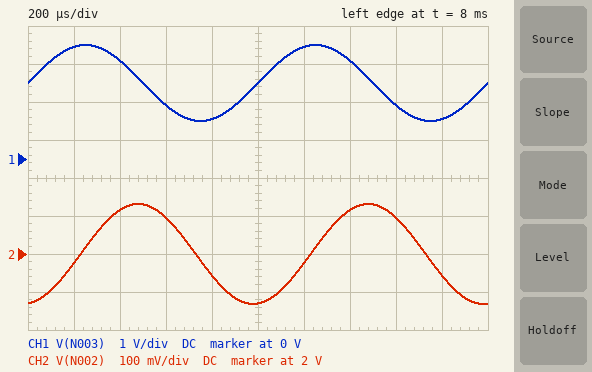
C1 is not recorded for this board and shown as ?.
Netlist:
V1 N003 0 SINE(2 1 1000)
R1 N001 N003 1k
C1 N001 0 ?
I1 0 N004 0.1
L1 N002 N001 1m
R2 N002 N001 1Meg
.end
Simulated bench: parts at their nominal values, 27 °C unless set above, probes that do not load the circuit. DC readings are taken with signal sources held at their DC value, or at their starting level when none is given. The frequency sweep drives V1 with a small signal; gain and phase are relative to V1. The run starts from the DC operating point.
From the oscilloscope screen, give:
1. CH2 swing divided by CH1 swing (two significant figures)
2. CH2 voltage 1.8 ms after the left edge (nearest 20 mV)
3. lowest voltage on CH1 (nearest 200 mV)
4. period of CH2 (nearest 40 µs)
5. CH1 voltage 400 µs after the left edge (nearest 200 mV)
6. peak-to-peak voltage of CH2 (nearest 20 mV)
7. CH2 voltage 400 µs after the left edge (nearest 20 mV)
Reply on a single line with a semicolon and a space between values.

0.13; 1.94 V; 1.0 V; 1.00 ms; 2.6 V; 260 mV; 2.12 V
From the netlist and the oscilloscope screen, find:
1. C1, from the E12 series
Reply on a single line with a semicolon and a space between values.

1.2 µF
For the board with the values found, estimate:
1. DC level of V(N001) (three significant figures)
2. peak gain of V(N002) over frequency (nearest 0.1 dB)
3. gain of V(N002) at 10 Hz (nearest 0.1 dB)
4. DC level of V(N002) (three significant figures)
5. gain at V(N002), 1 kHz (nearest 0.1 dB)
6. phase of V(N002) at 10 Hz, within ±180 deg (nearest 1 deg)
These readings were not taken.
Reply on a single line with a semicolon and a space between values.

2.00 V; 0 dB; 0 dB; 2.00 V; -17.6 dB; -4 deg
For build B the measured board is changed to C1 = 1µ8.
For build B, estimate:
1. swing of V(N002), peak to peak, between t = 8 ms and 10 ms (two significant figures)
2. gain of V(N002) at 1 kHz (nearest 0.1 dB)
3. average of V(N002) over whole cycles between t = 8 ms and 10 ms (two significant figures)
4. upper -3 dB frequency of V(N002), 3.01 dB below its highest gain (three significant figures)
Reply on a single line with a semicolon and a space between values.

180 mV; -21.1 dB; 2.0 V; 88.4 Hz
